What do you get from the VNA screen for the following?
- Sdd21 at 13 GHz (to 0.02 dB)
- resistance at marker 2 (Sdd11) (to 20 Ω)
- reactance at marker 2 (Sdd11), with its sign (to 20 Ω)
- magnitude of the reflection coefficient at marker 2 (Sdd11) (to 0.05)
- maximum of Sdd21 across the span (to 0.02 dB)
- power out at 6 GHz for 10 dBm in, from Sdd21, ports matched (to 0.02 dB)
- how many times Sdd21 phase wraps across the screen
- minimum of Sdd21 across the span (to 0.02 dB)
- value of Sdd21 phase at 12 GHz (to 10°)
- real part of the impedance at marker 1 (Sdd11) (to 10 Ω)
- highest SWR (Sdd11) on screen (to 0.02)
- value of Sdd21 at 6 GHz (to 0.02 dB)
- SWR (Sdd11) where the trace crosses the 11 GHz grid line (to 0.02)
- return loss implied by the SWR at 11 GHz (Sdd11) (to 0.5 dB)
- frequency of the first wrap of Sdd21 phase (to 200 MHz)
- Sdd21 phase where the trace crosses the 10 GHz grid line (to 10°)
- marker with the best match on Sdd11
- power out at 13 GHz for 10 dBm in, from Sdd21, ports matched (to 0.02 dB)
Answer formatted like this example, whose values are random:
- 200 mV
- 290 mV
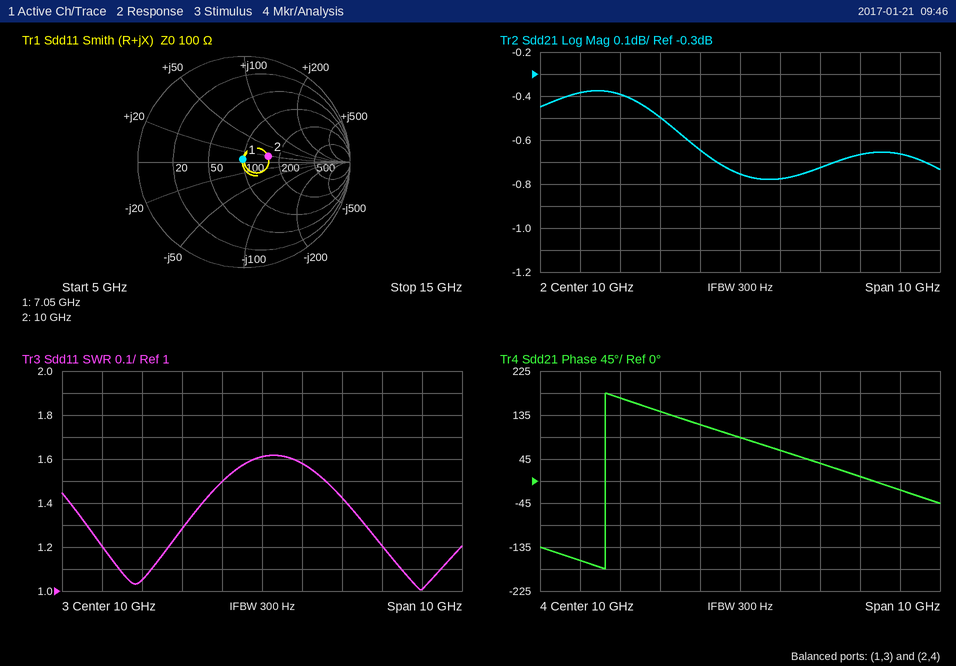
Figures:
- -0.66 dB
- 160 Ω
- +20 Ω
- 0.25
- -0.38 dB
- 9.62 dBm
- 1
- -0.78 dB
- 40°
- 100 Ω
- 1.62
- -0.38 dB
- 1.58
- 13.0 dB
- 6.6 GHz
- 90°
- marker 1
- 9.34 dBm
